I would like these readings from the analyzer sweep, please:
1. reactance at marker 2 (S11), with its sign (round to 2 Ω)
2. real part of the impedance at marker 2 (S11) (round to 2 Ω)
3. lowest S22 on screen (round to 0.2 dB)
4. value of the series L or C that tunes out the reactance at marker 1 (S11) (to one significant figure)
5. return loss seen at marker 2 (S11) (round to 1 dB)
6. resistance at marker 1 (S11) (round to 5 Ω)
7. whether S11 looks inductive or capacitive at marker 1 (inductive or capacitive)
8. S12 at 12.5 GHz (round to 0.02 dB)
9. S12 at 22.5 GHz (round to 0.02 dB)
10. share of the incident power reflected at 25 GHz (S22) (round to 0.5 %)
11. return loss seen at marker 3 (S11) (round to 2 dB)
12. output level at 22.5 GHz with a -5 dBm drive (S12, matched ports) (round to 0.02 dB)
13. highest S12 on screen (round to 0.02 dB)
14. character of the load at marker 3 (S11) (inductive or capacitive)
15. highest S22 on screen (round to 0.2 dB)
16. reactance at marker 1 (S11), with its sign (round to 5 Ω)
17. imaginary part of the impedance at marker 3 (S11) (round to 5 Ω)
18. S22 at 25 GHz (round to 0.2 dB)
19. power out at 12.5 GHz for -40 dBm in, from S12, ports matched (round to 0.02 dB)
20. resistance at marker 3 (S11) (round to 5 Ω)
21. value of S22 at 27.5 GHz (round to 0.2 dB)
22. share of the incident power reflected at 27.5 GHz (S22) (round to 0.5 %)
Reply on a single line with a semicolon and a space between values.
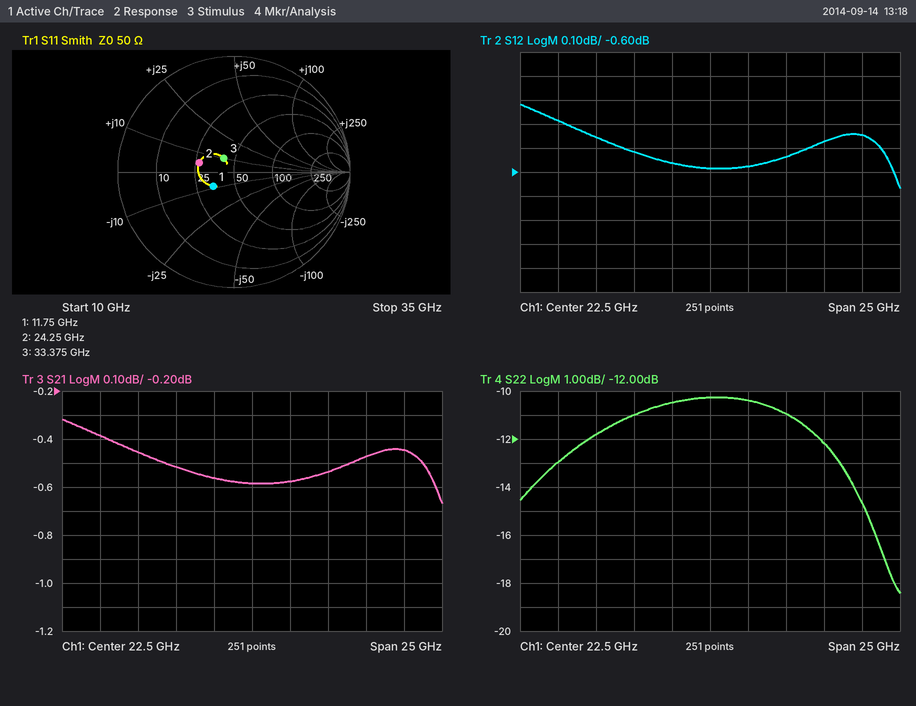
+4 Ω; 26 Ω; -18.4 dB; 100 pH; 10 dB; 35 Ω; capacitive; -0.38 dB; -0.58 dB; 9.0 %; 16 dB; -5.58 dBm; -0.32 dB; inductive; -10.2 dB; -10 Ω; +10 Ω; -10.4 dB; -40.38 dBm; 40 Ω; -11.0 dB; 8.0 %
